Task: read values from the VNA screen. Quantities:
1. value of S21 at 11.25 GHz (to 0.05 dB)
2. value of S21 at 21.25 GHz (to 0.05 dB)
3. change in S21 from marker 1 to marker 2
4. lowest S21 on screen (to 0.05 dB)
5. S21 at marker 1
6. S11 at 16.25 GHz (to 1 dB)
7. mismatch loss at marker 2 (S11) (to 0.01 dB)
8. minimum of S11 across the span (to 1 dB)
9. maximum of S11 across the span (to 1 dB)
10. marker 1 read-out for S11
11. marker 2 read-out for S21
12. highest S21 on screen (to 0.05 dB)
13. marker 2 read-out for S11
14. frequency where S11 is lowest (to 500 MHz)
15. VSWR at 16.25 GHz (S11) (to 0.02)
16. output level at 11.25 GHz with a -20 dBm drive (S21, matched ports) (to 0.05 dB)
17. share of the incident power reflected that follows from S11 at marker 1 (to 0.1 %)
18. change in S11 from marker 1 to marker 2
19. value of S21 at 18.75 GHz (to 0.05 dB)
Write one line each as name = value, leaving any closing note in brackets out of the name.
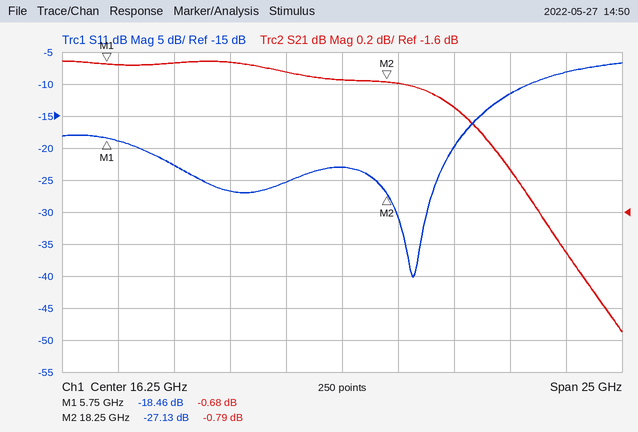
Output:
value of S21 at 11.25 GHz = -0.65 dB
value of S21 at 21.25 GHz = -0.95 dB
change in S21 from marker 1 to marker 2 = -0.11 dB
lowest S21 on screen = -2.35 dB
S21 at marker 1 = -0.68 dB
S11 at 16.25 GHz = -23 dB
mismatch loss at marker 2 (S11) = 0.01 dB
minimum of S11 across the span = -40 dB
maximum of S11 across the span = -7 dB
marker 1 read-out for S11 = -18.46 dB
marker 2 read-out for S21 = -0.79 dB
highest S21 on screen = -0.65 dB
marker 2 read-out for S11 = -27.13 dB
frequency where S11 is lowest = 19.5 GHz
VSWR at 16.25 GHz (S11) = 1.16
output level at 11.25 GHz with a -20 dBm drive (S21, matched ports) = -20.65 dBm
share of the incident power reflected that follows from S11 at marker 1 = 1.4 %
change in S11 from marker 1 to marker 2 = -8.67 dB
value of S21 at 18.75 GHz = -0.80 dB
